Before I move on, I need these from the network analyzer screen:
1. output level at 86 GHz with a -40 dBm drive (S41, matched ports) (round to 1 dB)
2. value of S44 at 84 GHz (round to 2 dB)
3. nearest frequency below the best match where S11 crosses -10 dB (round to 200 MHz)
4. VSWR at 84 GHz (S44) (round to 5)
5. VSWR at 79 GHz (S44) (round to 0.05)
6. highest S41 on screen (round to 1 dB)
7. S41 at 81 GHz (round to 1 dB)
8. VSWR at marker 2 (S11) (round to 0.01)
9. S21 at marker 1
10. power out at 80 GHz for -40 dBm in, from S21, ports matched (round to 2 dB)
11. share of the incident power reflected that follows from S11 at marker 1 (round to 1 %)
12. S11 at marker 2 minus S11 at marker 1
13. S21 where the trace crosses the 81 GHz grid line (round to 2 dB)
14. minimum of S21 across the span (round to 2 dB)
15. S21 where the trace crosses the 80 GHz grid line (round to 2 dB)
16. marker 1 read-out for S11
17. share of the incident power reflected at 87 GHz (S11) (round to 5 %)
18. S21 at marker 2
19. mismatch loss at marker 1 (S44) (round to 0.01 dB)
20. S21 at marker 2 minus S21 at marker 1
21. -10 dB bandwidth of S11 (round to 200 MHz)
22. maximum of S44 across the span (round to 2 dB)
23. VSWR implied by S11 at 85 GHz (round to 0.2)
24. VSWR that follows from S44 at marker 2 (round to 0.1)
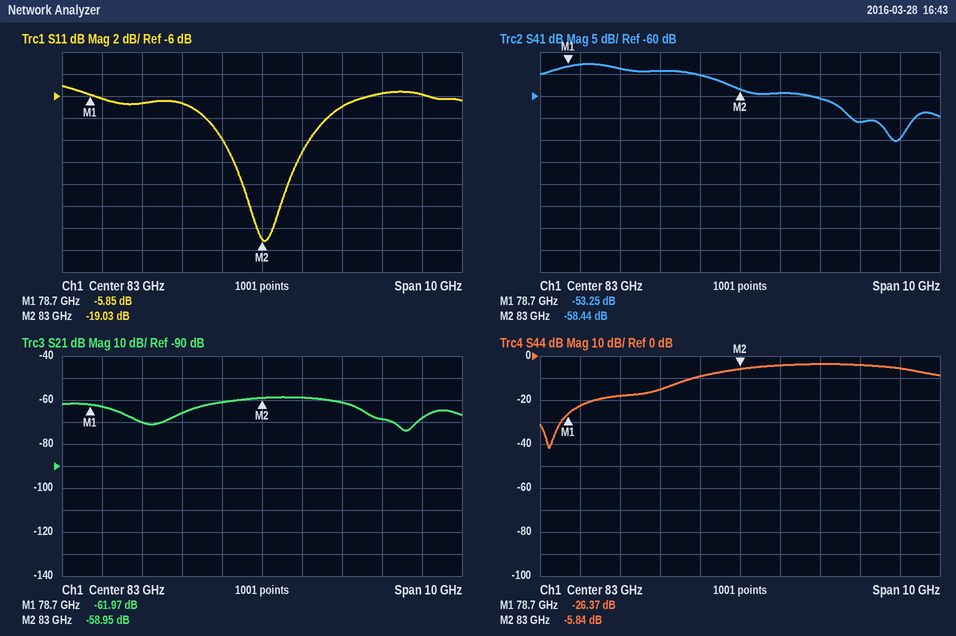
-106 dBm
-4 dB
82.0 GHz
5
1.15
-53 dB
-54 dB
1.25
-61.97 dB
-110 dBm
26 %
-13.18 dB
-66 dB
-74 dB
-70 dB
-5.85 dB
25 %
-58.95 dB
0.01 dB
3.02 dB
2.2 GHz
-4 dB
2.6
3.1
